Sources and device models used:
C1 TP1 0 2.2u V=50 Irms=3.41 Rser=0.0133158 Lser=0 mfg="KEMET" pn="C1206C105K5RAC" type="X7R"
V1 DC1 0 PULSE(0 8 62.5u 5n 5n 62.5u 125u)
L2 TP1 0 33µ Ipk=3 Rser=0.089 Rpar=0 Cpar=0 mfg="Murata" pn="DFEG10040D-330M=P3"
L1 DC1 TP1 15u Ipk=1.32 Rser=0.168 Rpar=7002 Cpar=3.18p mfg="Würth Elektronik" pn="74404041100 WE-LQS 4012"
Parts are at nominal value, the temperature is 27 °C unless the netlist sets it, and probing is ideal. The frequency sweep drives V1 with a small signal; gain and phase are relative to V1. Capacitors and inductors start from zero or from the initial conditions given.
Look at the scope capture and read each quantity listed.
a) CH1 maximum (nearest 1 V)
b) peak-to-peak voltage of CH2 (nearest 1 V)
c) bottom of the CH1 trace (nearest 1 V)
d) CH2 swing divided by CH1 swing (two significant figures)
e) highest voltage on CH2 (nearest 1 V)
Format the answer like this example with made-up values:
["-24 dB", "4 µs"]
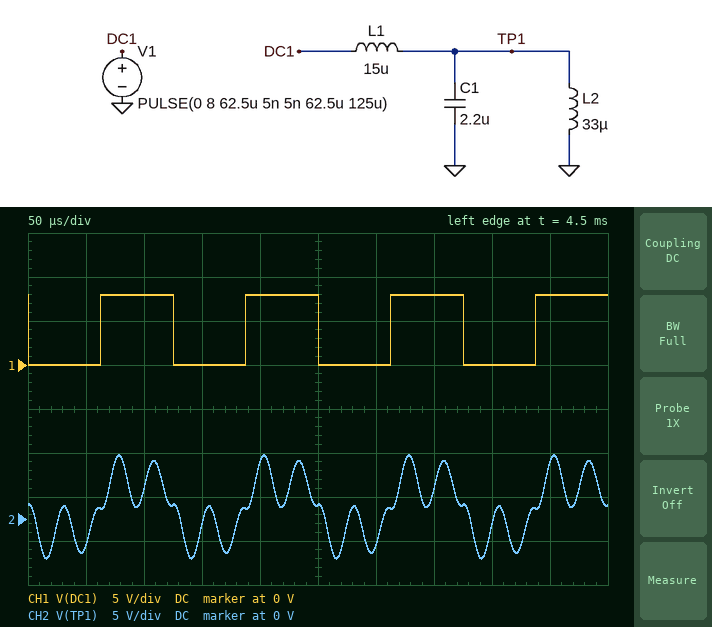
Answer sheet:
["8 V", "12 V", "0 V", "1.5", "7 V"]
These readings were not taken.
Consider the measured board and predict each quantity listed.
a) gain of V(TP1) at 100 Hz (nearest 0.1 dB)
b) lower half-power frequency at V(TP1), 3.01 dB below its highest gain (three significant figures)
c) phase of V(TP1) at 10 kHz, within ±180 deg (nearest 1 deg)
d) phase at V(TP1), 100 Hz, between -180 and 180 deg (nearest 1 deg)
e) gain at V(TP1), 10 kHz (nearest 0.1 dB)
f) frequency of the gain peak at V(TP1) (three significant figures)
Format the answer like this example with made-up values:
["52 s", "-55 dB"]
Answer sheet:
["-9.0 dB", "32.6 kHz", "2 deg", "6 deg", "-2.5 dB", "33.4 kHz"]
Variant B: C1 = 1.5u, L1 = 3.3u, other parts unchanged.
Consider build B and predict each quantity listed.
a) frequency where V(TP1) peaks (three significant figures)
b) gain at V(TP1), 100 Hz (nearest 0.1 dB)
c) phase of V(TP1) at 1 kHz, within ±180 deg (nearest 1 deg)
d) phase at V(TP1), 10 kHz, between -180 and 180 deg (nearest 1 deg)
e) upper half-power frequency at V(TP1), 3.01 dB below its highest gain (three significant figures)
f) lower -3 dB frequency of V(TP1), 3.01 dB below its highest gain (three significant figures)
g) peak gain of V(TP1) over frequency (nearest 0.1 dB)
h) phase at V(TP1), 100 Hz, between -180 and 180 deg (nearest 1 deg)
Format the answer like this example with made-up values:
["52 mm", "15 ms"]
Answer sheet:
["74.8 kHz", "-9.0 dB", "25 deg", "3 deg", "78.7 kHz", "70.6 kHz", "18.5 dB", "8 deg"]
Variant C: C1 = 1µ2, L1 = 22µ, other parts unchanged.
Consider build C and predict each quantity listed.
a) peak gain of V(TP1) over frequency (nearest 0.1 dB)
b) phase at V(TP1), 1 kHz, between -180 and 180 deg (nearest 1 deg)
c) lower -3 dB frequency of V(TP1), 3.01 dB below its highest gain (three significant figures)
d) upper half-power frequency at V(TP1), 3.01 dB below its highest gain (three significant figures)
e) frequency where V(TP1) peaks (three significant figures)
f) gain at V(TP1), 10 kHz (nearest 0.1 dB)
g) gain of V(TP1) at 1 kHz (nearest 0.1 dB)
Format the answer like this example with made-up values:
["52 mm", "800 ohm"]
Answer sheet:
["26.9 dB", "13 deg", "39.4 kHz", "40.5 kHz", "40.0 kHz", "-3.9 dB", "-5.6 dB"]
